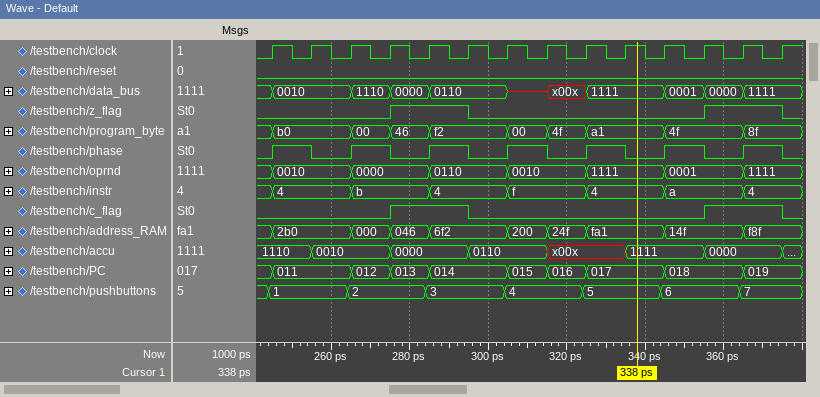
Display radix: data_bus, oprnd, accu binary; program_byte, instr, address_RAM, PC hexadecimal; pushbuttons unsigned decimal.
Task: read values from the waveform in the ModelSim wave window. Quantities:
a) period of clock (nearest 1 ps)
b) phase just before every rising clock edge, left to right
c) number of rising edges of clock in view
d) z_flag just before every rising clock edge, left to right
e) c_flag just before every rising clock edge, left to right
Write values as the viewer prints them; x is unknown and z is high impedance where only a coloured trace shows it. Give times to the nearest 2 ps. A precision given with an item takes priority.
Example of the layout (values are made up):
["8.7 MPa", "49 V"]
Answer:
["10 ps", "0 1 0 1 0 1 0 1 0 1 0 1 0 1", "14", "0 0 0 0 1 1 0 0 0 0 0 0 1 1", "0 0 0 0 1 1 0 0 0 0 0 0 1 1"]
